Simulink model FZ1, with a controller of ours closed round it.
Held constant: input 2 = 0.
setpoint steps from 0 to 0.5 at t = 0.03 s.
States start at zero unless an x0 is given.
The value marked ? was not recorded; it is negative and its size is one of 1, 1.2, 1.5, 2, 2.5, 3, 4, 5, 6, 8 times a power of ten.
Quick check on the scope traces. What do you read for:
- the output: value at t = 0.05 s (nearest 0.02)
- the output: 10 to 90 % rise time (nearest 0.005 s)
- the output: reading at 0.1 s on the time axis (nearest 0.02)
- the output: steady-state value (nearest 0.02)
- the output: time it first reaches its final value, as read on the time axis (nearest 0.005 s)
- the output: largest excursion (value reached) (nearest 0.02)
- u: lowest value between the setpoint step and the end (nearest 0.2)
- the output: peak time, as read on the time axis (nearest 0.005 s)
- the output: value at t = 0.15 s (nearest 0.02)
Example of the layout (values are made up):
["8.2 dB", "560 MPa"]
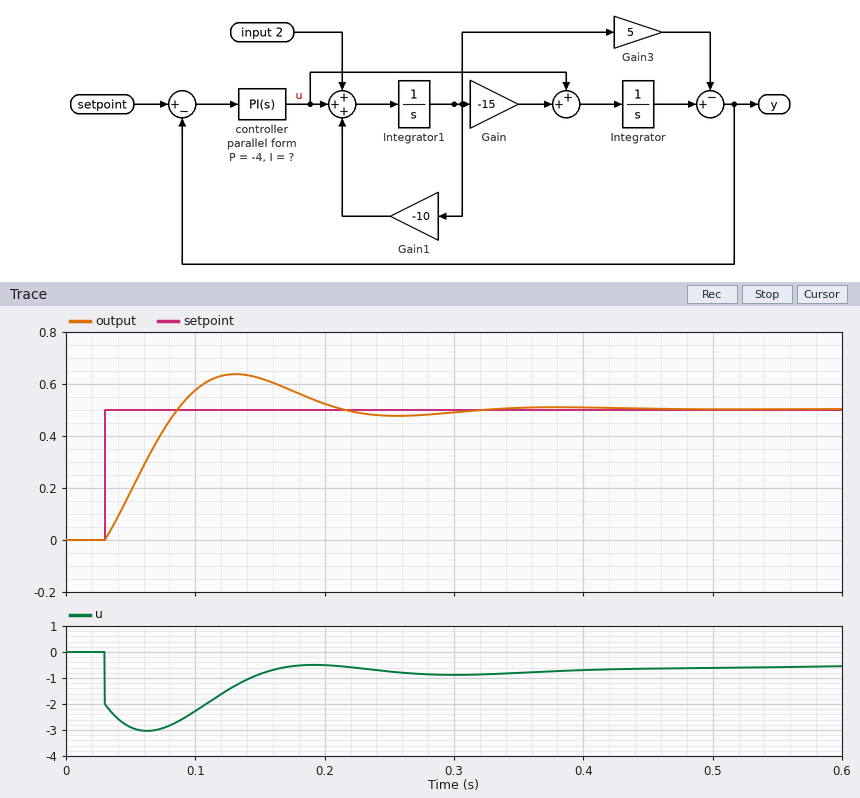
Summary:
["0.18", "0.045 s", "0.58", "0.50", "0.085 s", "0.64", "-3.0", "0.130 s", "0.62"]
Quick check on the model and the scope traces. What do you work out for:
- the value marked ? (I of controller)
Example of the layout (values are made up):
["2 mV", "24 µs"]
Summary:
["-200"]
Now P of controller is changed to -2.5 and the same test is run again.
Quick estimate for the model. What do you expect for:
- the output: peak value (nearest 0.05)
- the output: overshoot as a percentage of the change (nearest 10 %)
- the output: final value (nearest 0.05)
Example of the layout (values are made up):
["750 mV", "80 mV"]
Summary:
["0.70", "40 %", "0.50"]
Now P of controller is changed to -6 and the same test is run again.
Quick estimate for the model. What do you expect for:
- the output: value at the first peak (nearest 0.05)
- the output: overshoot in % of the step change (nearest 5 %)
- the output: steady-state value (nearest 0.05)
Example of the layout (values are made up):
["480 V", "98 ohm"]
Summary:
["0.60", "20 %", "0.50"]
